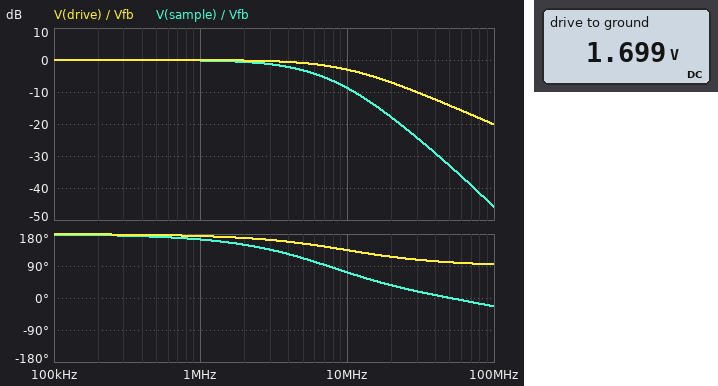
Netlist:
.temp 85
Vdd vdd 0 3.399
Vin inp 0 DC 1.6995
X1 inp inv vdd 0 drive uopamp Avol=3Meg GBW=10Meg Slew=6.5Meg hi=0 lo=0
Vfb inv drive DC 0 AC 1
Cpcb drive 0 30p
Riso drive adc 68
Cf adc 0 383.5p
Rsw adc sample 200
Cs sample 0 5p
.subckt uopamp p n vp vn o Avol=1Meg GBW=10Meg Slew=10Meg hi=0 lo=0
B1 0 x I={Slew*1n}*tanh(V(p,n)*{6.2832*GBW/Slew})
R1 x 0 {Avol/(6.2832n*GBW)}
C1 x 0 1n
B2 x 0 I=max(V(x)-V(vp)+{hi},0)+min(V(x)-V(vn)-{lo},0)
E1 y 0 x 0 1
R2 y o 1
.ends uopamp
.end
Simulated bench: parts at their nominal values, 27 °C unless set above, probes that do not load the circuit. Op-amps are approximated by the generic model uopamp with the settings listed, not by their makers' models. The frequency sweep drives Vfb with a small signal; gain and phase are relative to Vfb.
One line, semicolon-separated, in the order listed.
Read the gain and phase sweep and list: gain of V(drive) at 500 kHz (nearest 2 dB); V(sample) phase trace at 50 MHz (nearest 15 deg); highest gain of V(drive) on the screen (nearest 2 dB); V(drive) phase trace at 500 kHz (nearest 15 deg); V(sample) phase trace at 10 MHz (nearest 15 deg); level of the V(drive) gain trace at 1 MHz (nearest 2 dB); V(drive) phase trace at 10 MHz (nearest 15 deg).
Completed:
0 dB; 0 deg; 0 dB; 180 deg; 75 deg; 0 dB; 135 deg
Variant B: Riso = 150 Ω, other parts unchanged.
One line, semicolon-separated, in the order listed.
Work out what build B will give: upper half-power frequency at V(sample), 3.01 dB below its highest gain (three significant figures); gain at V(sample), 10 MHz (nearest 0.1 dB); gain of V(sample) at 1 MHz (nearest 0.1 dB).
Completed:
2.56 MHz; -14.6 dB; -0.6 dB
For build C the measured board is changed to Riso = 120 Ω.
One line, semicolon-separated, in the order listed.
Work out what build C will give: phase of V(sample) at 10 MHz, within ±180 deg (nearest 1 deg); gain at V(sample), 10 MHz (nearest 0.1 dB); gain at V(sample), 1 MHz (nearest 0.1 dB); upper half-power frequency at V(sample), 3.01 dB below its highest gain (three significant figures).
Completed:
60 deg; -12.9 dB; -0.4 dB; 3.10 MHz
